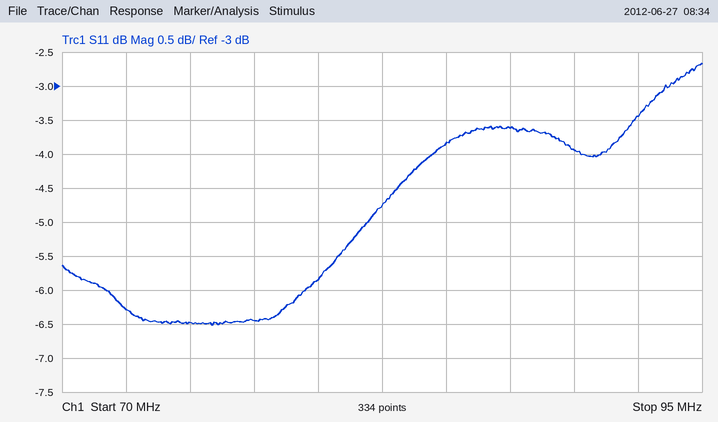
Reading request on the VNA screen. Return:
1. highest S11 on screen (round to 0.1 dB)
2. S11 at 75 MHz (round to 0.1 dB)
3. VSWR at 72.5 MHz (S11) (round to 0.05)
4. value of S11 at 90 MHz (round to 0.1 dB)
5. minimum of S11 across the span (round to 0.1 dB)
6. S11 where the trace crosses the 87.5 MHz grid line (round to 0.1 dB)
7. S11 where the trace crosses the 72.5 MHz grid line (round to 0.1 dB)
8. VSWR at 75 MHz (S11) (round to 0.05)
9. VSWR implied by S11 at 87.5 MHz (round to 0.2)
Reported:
-2.7 dB
-6.5 dB
2.90
-3.9 dB
-6.5 dB
-3.6 dB
-6.3 dB
2.80
4.8
